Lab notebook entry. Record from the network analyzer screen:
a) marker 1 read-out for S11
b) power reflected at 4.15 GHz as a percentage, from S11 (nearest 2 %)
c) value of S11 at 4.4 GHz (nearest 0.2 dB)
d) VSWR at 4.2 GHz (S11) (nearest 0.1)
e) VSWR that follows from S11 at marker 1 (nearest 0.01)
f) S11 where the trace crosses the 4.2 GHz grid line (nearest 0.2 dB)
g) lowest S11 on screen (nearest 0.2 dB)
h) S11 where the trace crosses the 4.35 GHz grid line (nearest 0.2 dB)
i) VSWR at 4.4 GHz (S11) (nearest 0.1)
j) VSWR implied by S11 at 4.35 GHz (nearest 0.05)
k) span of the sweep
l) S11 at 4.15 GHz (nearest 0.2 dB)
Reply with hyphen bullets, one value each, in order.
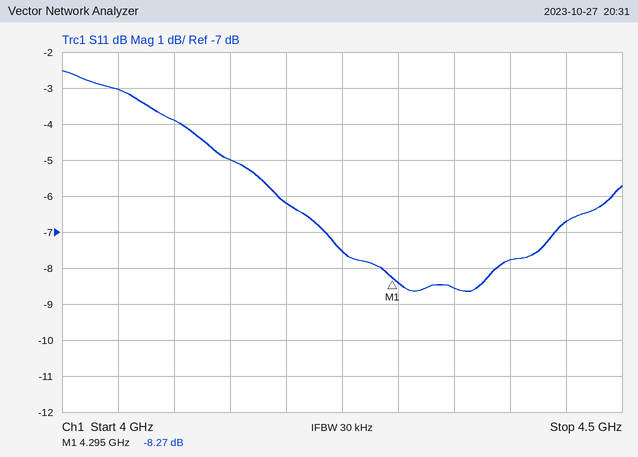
- -8.27 dB
- 32 %
- -7.8 dB
- 2.9
- 2.26
- -6.2 dB
- -8.6 dB
- -8.6 dB
- 2.4
- 2.20
- 500 MHz
- -5.0 dB
